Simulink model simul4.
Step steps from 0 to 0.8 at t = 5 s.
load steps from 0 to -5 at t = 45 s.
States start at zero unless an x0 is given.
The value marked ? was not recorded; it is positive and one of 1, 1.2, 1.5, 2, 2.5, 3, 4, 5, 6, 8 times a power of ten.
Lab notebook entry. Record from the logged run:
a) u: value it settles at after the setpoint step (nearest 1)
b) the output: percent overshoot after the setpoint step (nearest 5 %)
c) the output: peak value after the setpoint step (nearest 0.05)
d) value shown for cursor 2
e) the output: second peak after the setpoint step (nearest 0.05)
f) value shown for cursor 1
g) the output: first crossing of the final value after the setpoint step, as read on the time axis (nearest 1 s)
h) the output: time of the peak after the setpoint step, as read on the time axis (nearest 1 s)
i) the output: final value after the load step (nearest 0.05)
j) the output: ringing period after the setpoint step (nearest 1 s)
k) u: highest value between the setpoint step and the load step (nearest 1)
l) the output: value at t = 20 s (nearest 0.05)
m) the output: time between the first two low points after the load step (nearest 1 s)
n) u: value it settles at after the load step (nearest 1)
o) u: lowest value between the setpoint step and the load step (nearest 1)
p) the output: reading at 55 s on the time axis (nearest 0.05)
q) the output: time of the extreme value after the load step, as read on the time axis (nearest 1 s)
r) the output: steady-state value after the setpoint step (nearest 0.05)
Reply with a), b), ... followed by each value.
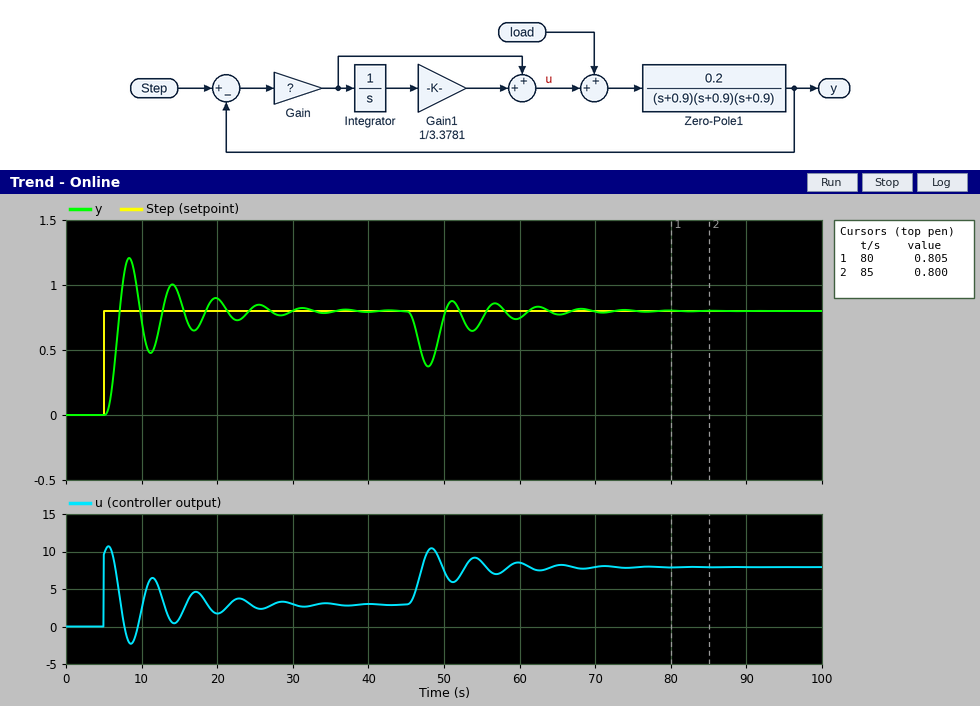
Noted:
a) 3
b) 50 %
c) 1.20
d) 0.800
e) 1.00
f) 0.805
g) 7 s
h) 8 s
i) 0.80
j) 6 s
k) 11
l) 0.90
m) 6 s
n) 8
o) -2
p) 0.75
q) 48 s
r) 0.80
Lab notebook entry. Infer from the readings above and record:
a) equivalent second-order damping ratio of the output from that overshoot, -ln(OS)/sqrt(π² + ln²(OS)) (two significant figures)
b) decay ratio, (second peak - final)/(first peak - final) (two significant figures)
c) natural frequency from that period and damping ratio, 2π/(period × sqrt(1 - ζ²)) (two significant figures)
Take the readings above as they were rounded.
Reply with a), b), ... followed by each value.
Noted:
a) 0.22
b) 0.50
c) 1.1 rad/s
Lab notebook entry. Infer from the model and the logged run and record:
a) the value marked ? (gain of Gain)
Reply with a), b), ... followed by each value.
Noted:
a) 12
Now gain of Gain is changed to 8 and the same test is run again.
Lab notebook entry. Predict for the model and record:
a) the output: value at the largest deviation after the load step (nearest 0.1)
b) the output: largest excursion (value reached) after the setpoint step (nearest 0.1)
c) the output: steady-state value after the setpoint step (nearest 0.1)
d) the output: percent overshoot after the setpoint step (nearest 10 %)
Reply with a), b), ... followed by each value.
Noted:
a) 0.3
b) 1.0
c) 0.8
d) 30 %
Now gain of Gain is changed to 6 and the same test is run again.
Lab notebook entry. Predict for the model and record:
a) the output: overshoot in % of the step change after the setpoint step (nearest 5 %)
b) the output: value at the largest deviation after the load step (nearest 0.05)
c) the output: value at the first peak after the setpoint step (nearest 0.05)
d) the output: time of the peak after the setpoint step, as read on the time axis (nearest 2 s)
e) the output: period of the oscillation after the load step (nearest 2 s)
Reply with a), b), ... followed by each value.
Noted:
a) 15 %
b) 0.20
c) 0.95
d) 10 s
e) 8 s
